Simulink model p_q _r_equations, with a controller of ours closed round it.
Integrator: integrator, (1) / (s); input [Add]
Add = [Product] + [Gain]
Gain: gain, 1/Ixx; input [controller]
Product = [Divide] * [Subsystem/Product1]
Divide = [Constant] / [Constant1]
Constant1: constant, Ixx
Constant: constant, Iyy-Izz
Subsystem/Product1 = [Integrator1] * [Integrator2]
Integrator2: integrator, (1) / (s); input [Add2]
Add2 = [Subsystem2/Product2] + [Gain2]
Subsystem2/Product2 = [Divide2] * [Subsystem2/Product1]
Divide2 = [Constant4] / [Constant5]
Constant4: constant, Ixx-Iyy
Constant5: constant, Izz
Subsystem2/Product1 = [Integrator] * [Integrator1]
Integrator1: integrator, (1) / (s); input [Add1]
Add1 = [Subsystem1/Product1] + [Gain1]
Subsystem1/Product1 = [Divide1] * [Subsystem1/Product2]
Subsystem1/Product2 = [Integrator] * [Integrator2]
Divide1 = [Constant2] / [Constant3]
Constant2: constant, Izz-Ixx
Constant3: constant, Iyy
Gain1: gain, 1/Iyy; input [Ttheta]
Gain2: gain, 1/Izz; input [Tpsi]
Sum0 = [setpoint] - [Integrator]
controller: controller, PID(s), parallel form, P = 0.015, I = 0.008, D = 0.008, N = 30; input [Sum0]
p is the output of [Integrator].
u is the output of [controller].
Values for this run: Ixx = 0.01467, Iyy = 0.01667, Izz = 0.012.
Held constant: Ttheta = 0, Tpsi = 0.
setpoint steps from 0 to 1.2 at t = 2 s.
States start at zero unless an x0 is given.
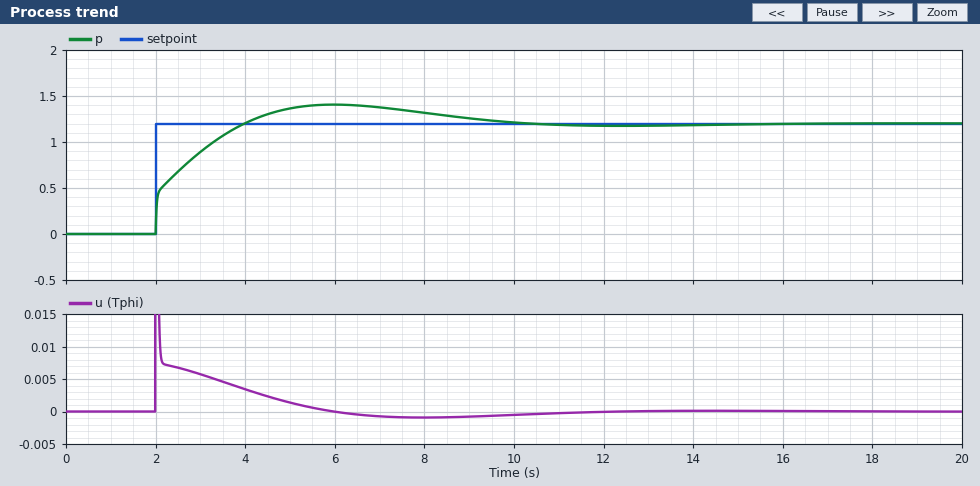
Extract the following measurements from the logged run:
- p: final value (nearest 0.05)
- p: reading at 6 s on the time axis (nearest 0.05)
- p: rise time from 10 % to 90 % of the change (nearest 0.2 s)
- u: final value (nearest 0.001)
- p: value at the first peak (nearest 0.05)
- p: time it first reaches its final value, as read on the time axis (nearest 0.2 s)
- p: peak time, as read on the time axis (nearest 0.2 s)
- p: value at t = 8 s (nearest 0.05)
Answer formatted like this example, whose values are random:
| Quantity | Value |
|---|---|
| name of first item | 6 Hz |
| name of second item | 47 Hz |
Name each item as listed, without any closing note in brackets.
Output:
| Quantity | Value |
|---|---|
| p: final value | 1.20 |
| p: reading at 6 s on the time axis | 1.40 |
| p: rise time from 10 % to 90 % of the change | 1.6 s |
| u: final value | 0.000 |
| p: value at the first peak | 1.40 |
| p: time it first reaches its final value, as read on the time axis | 4.0 s |
| p: peak time, as read on the time axis | 6.0 s |
| p: value at t = 8 s | 1.30 |
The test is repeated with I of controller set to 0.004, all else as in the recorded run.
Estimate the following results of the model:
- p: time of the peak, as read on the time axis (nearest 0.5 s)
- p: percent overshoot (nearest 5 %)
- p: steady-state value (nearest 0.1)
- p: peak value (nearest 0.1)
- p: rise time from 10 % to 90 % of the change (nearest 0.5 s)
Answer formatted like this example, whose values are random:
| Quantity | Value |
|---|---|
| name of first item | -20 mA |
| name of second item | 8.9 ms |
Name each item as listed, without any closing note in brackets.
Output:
| Quantity | Value |
|---|---|
| p: time of the peak, as read on the time axis | 7.0 s |
| p: percent overshoot | 10 % |
| p: steady-state value | 1.2 |
| p: peak value | 1.3 |
| p: rise time from 10 % to 90 % of the change | 2.0 s |
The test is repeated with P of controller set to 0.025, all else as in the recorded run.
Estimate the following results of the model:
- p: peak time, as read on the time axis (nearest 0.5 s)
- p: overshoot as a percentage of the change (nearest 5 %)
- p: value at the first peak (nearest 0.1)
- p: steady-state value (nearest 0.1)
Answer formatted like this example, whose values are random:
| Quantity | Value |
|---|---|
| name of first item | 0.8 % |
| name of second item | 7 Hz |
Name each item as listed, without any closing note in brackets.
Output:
| Quantity | Value |
|---|---|
| p: peak time, as read on the time axis | 5.5 s |
| p: overshoot as a percentage of the change | 10 % |
| p: value at the first peak | 1.3 |
| p: steady-state value | 1.2 |
